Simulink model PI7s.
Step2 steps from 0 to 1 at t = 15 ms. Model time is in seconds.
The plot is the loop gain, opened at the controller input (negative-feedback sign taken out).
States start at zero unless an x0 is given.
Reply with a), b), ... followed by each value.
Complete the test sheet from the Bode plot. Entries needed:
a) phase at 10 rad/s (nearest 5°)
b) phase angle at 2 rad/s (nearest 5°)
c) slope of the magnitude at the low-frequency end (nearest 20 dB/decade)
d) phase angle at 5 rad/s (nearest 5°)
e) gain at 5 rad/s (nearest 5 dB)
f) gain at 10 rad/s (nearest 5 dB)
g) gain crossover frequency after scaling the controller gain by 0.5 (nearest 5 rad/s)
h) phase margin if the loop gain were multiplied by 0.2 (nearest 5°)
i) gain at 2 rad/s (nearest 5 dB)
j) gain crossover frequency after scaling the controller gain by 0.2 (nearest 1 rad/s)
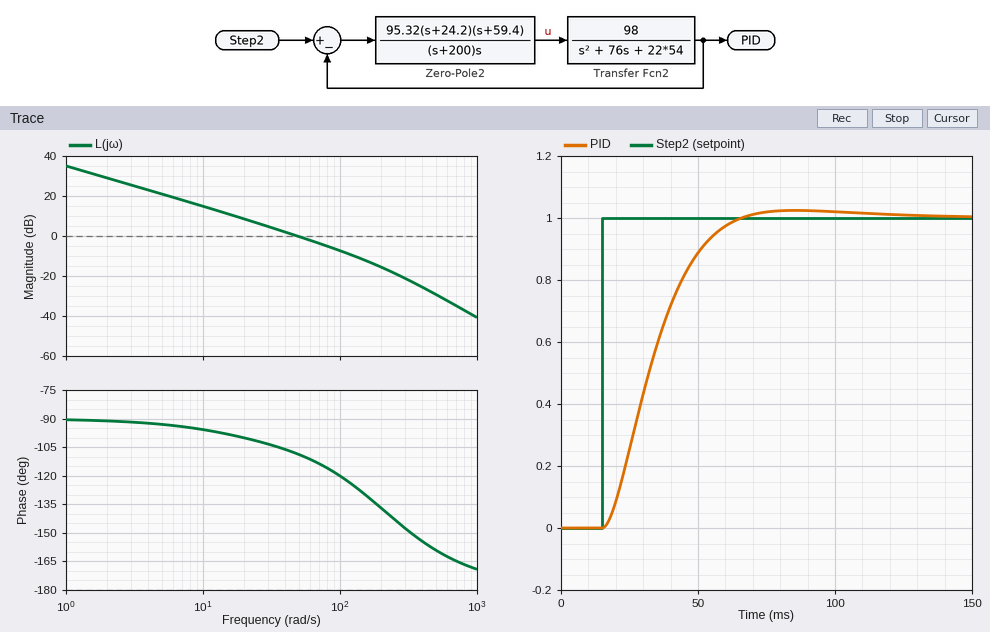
a) -95°
b) -90°
c) -20 dB/decade
d) -95°
e) 20 dB
f) 15 dB
g) 25 rad/s
h) 85°
i) 30 dB
j) 11 rad/s
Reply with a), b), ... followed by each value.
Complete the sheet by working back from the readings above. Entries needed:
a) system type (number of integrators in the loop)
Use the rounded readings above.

a) 1
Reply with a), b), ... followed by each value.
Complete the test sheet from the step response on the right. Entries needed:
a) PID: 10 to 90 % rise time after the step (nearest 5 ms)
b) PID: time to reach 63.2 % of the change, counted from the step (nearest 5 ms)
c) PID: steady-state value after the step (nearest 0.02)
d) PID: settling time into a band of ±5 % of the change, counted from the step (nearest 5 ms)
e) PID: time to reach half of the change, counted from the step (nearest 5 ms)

a) 30 ms
b) 20 ms
c) 1.00
d) 40 ms
e) 15 ms
